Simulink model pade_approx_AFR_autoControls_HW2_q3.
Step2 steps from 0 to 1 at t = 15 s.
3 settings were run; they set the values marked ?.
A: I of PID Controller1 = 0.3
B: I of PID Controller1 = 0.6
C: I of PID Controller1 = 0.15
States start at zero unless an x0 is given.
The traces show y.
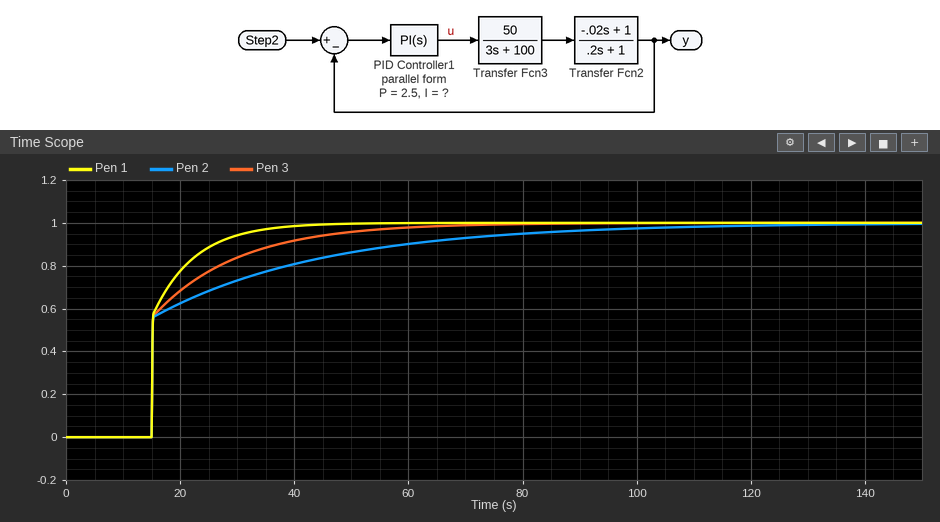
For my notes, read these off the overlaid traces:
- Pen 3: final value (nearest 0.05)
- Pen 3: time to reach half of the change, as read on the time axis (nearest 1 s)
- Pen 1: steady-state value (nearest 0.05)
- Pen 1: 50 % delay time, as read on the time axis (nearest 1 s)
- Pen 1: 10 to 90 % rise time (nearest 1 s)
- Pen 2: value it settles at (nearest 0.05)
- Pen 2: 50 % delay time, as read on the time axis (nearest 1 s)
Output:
1.00
15 s
1.00
15 s
11 s
1.00
15 s
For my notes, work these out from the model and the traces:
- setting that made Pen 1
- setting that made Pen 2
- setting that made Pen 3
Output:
B
C
A
